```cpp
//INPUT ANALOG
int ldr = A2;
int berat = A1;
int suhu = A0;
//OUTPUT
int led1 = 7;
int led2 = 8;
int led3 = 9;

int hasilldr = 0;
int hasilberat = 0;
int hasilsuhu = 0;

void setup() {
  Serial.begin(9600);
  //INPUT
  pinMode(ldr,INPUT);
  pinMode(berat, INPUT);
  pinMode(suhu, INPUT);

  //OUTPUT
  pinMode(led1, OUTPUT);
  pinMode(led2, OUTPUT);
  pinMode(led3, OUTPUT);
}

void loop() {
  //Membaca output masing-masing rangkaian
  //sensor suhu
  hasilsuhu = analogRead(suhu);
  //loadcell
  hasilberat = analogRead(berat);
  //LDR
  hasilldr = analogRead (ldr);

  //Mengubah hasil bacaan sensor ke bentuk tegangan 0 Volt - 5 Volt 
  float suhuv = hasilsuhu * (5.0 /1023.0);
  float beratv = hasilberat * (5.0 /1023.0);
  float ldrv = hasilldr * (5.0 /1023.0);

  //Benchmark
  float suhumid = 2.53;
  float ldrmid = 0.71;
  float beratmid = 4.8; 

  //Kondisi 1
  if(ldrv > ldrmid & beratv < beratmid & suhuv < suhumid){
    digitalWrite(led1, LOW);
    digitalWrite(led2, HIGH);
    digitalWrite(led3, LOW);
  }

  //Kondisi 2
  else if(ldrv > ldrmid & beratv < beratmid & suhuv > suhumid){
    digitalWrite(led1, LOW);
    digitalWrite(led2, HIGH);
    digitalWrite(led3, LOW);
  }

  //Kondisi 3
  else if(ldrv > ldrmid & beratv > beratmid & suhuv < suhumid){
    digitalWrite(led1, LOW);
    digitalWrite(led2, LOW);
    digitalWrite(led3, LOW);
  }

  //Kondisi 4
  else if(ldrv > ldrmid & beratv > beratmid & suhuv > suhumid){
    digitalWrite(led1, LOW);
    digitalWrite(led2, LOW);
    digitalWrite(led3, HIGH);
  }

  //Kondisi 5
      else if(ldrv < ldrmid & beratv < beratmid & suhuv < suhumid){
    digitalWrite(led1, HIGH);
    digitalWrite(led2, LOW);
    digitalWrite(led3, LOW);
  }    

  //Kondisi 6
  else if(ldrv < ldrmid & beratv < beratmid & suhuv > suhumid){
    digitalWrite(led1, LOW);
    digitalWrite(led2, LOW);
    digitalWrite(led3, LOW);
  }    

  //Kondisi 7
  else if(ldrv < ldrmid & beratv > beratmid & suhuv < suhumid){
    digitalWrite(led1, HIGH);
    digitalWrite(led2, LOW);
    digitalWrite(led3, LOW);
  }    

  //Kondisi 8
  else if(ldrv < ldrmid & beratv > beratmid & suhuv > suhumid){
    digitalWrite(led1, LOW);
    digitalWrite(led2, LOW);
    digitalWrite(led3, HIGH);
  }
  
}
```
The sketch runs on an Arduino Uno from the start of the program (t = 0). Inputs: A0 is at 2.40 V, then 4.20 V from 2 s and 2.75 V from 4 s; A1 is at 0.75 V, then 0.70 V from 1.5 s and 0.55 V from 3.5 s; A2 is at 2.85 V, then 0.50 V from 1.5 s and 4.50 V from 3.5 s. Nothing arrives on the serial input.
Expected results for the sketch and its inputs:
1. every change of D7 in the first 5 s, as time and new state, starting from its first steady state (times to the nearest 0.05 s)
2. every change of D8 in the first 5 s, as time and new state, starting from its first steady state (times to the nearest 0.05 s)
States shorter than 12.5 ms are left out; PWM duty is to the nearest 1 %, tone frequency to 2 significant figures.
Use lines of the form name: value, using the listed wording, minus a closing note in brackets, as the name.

every change of D7 in the first 5 s, as time and new state, starting from its first steady state: 0 s low; 1.5 s high; 2 s low
every change of D8 in the first 5 s, as time and new state, starting from its first steady state: 0 s high; 1.5 s low; 3.5 s high
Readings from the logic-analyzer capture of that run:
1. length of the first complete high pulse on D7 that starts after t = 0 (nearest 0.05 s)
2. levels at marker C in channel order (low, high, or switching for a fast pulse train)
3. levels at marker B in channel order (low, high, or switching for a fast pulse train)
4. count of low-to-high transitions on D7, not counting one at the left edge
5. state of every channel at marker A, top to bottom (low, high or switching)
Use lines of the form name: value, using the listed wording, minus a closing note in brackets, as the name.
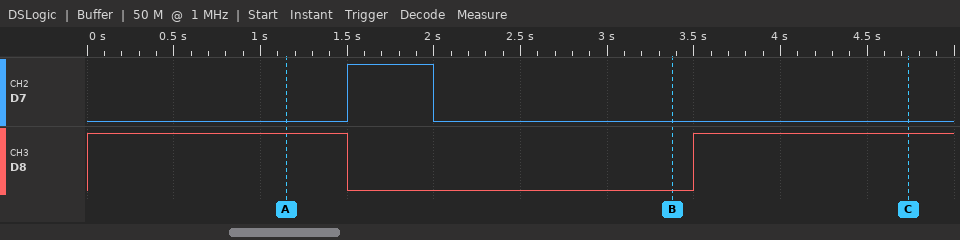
length of the first complete high pulse on D7 that starts after t = 0: 0.50 s
levels at marker C in channel order: D7 low, D8 high
levels at marker B in channel order: D7 low, D8 low
count of low-to-high transitions on D7, not counting one at the left edge: 1
state of every channel at marker A, top to bottom: D7 low, D8 high
